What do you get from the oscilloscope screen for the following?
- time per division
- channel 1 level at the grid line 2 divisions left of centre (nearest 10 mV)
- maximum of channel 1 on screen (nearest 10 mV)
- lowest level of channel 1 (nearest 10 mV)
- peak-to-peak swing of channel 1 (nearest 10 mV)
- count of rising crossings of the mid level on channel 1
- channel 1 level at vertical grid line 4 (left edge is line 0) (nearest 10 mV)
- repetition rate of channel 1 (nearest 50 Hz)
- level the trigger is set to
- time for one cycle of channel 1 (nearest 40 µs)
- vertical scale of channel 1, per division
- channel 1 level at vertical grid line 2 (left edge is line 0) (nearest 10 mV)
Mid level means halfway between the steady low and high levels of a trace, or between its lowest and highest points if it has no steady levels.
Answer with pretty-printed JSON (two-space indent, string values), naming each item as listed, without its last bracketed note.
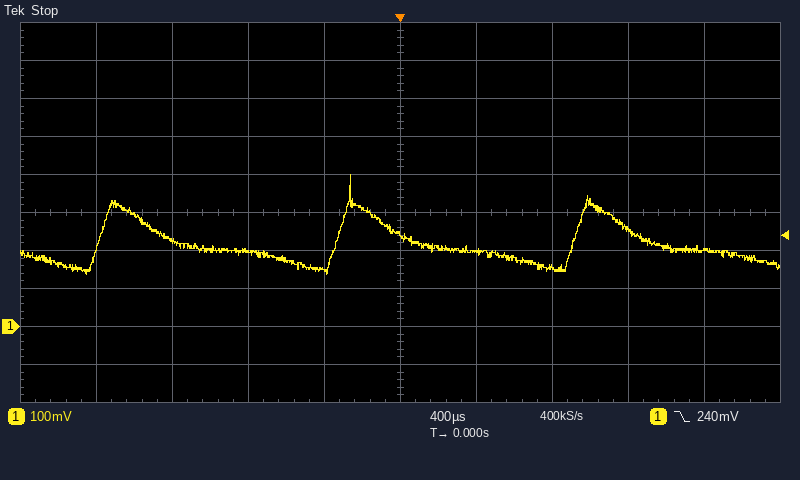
{
  "time per division": "400 µs",
  "channel 1 level at the grid line 2 divisions left of centre": "200 mV",
  "maximum of channel 1 on screen": "400 mV",
  "lowest level of channel 1": "140 mV",
  "peak-to-peak swing of channel 1": "260 mV",
  "count of rising crossings of the mid level on channel 1": "3",
  "channel 1 level at vertical grid line 4 (left edge is line 0)": "150 mV",
  "repetition rate of channel 1": "800 Hz",
  "level the trigger is set to": "240 mV",
  "time for one cycle of channel 1": "1.24 ms",
  "vertical scale of channel 1, per division": "100 mV",
  "channel 1 level at vertical grid line 2 (left edge is line 0)": "230 mV"
}
